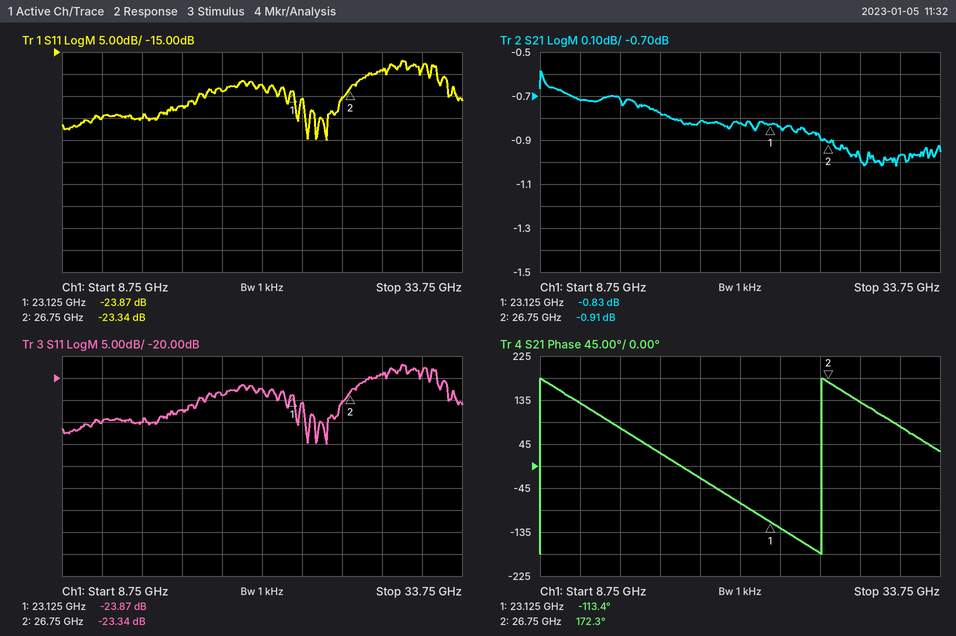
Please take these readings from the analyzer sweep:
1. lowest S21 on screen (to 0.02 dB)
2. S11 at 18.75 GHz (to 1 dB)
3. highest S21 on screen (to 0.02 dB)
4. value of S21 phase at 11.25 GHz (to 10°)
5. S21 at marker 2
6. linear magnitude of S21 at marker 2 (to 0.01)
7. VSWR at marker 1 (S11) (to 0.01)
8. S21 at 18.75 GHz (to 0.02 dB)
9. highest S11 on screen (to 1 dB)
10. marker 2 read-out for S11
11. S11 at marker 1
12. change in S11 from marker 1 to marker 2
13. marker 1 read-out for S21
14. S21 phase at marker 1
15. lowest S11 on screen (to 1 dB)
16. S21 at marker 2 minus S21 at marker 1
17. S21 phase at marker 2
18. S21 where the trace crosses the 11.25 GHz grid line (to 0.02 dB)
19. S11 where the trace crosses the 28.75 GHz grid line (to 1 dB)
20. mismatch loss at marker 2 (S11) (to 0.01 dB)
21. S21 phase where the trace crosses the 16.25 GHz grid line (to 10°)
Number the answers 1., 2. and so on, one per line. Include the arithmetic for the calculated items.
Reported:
1. -1.02 dB
2. -24 dB
3. -0.58 dB
4. 130°
5. -0.91 dB
6. 10^(-0.91/20) ≈ 0.90
7. (1 + 0.0640)/(1 − 0.0640) ≈ 1.14
8. -0.82 dB
9. -17 dB
10. -23.34 dB
11. -23.87 dB
12. -23.34 − (-23.87) = 0.53 dB
13. -0.83 dB
14. -113.4°
15. -35 dB
16. -0.91 − (-0.83) = -0.08 dB
17. 172.3°
18. -0.72 dB
19. -19 dB
20. −10 log10(1 − 10^(-23.34/10)) ≈ 0.02 dB
21. 30°
